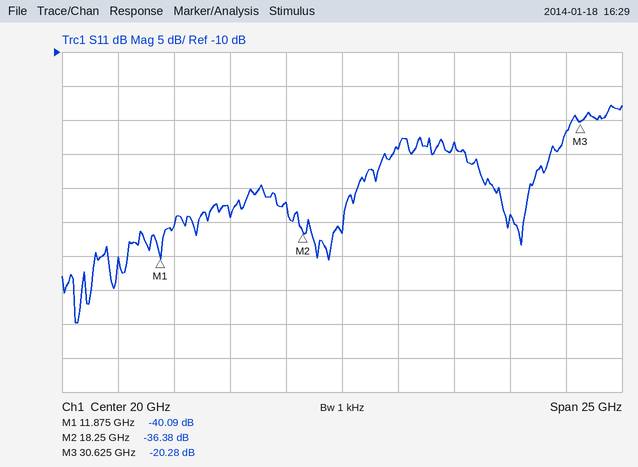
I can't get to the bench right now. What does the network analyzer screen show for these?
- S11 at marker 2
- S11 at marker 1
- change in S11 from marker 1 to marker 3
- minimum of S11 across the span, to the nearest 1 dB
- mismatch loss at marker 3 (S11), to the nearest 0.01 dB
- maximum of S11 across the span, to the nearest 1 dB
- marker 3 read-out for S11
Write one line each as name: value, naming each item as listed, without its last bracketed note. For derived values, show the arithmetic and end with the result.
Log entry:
S11 at marker 2: -36.38 dB
S11 at marker 1: -40.09 dB
change in S11 from marker 1 to marker 3: -20.28 − (-40.09) = 19.81 dB
minimum of S11 across the span, to the nearest 1 dB: -50 dB
mismatch loss at marker 3 (S11), to the nearest 0.01 dB: −10 log10(1 − 10^(-20.28/10)) ≈ 0.04 dB
maximum of S11 across the span, to the nearest 1 dB: -18 dB
marker 3 read-out for S11: -20.28 dB
